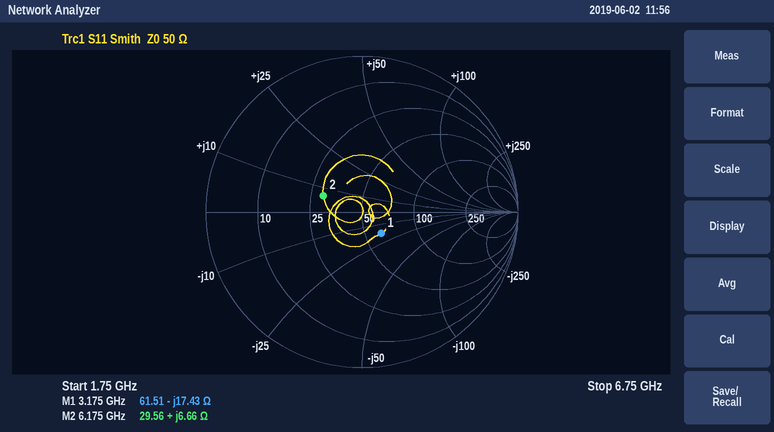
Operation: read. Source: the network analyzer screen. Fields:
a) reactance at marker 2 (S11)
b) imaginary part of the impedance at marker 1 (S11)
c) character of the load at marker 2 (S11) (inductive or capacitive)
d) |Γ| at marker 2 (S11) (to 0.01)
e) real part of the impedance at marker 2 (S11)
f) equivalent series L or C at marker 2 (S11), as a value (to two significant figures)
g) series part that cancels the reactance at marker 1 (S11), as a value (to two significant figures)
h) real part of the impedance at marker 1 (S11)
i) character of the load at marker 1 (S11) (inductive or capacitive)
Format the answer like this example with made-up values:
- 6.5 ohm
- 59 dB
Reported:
- +6.66 Ω
- -17.43 Ω
- inductive
- 0.27
- 29.56 Ω
- 170 pH
- 870 pH
- 61.51 Ω
- capacitive
